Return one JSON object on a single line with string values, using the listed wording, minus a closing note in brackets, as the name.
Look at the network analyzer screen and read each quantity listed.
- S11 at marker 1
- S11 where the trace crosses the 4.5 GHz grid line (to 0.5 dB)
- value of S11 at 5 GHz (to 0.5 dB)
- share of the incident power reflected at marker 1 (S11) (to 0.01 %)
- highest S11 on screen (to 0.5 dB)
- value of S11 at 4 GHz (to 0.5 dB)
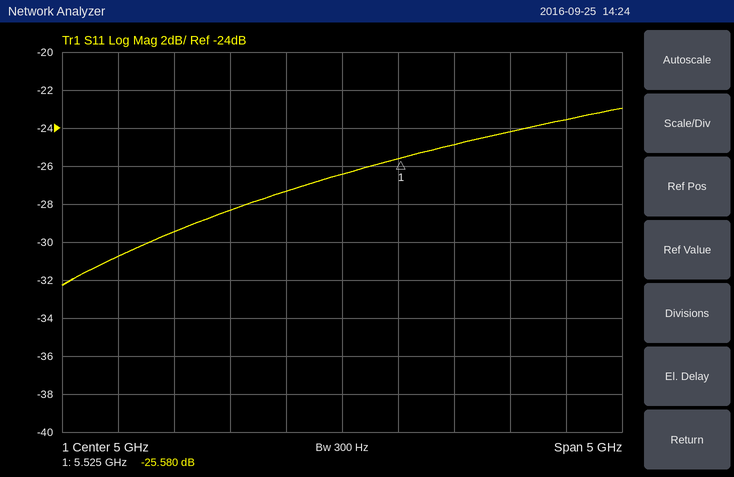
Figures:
{"S11 at marker 1": "-25.580 dB", "S11 where the trace crosses the 4.5 GHz grid line": "-27.5 dB", "value of S11 at 5 GHz": "-26.5 dB", "share of the incident power reflected at marker 1 (S11)": "0.28 %", "highest S11 on screen": "-23.0 dB", "value of S11 at 4 GHz": "-28.5 dB"}
